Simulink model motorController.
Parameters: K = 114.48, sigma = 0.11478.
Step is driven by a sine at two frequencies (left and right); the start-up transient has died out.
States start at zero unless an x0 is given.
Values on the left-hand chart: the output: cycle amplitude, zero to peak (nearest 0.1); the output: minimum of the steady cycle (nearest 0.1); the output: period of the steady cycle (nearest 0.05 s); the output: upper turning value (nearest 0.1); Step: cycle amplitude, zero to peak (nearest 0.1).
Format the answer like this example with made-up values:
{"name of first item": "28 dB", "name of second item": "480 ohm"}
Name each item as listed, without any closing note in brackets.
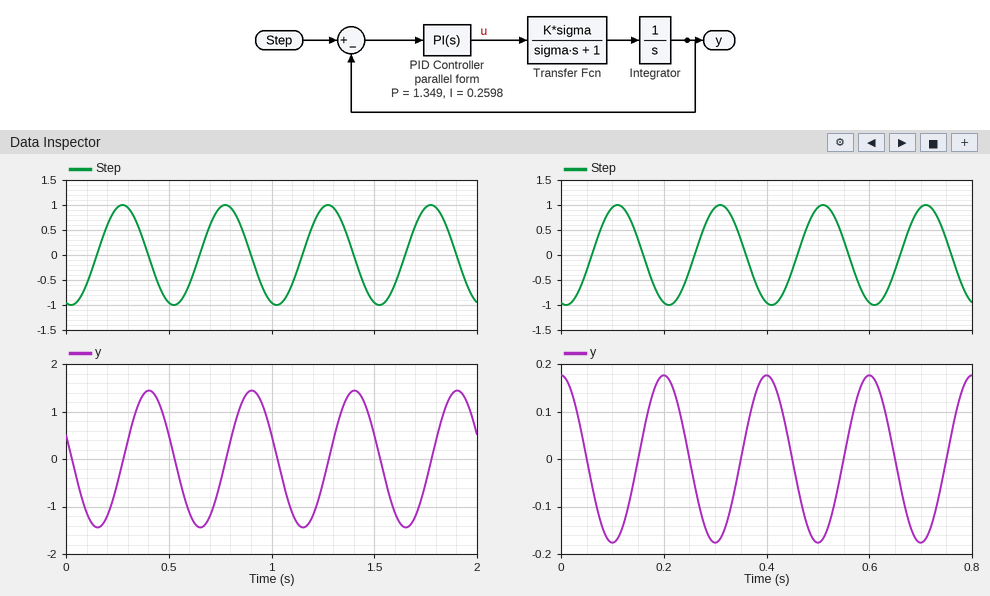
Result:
{"the output: cycle amplitude, zero to peak": "1.4", "the output: minimum of the steady cycle": "-1.4", "the output: period of the steady cycle": "0.50 s", "the output: upper turning value": "1.4", "Step: cycle amplitude, zero to peak": "1.0"}
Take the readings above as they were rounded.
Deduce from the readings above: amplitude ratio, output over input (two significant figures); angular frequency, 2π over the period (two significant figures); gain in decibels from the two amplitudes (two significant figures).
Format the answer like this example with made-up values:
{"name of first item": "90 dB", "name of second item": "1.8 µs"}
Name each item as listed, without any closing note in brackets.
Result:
{"amplitude ratio, output over input": "1.4", "angular frequency, 2π over the period": "13 rad/s", "gain in decibels from the two amplitudes": "2.9 dB"}
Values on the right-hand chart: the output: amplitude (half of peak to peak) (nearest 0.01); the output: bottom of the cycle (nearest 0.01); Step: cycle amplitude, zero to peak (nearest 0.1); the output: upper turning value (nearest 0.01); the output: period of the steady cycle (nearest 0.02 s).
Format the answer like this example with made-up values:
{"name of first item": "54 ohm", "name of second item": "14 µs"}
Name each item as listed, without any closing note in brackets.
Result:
{"the output: amplitude (half of peak to peak)": "0.18", "the output: bottom of the cycle": "-0.18", "Step: cycle amplitude, zero to peak": "1.0", "the output: upper turning value": "0.18", "the output: period of the steady cycle": "0.20 s"}
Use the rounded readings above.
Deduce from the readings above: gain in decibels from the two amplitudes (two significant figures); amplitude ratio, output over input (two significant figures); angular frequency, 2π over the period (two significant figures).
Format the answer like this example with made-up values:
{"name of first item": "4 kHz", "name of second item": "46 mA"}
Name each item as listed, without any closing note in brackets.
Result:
{"gain in decibels from the two amplitudes": "-15 dB", "amplitude ratio, output over input": "0.18", "angular frequency, 2π over the period": "31 rad/s"}
